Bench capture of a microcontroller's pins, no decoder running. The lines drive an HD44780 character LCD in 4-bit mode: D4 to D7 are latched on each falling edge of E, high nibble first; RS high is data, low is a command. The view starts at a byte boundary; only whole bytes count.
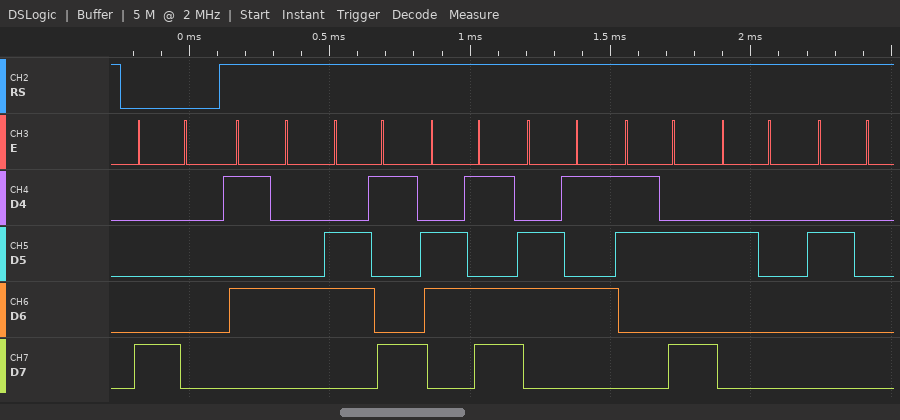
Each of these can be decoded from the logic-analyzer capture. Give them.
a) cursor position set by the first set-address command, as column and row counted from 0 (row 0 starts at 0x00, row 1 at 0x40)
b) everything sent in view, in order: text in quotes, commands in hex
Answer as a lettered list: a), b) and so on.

a) column 0, row 0
b) 0x80 "Time:  "
